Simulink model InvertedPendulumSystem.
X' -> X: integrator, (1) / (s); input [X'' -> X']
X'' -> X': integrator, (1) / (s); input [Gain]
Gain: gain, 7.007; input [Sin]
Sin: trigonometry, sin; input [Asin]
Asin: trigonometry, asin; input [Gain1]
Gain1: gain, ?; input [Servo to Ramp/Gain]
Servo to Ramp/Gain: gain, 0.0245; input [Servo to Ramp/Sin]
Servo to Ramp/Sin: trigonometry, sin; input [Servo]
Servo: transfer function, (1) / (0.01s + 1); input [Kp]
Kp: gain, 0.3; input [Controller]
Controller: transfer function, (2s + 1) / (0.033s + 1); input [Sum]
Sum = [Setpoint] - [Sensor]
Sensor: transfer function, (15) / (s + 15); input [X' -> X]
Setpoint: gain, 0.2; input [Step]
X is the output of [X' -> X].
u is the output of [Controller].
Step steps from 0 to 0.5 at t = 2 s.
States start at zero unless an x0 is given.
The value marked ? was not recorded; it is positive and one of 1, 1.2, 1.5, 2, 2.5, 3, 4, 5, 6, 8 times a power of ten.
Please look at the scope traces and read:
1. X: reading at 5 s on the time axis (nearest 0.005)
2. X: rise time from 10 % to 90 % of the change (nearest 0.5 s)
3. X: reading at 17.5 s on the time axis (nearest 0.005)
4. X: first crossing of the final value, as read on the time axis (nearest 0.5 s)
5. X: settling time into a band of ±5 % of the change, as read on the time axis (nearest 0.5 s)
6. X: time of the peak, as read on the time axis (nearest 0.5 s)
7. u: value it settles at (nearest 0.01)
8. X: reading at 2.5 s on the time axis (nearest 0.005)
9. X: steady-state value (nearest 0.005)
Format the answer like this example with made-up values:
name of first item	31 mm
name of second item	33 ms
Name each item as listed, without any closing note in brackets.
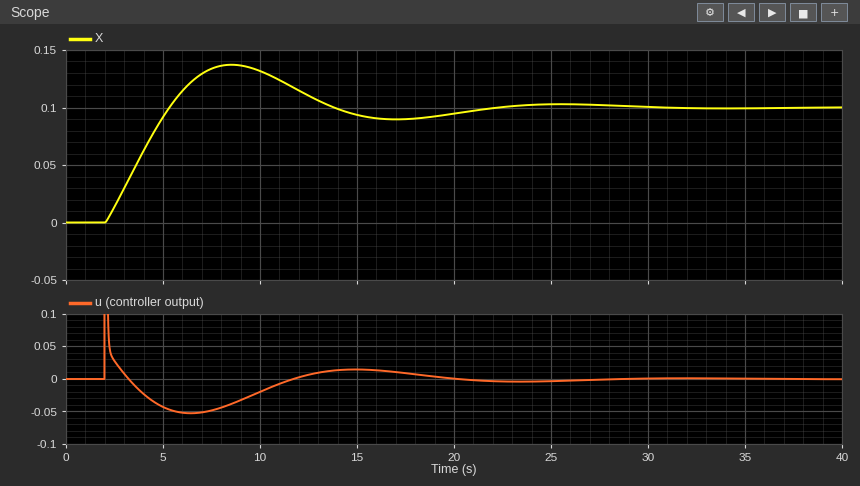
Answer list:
X: reading at 5 s on the time axis	0.090
X: rise time from 10 % to 90 % of the change	2.5 s
X: reading at 17.5 s on the time axis	0.090
X: first crossing of the final value, as read on the time axis	5.5 s
X: settling time into a band of ±5 % of the change, as read on the time axis	20.0 s
X: time of the peak, as read on the time axis	8.5 s
u: value it settles at	0.00
X: reading at 2.5 s on the time axis	0.015
X: steady-state value	0.100
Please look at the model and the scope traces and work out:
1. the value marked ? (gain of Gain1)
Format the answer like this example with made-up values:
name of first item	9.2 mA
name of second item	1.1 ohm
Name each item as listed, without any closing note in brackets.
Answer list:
the value marked ?	3
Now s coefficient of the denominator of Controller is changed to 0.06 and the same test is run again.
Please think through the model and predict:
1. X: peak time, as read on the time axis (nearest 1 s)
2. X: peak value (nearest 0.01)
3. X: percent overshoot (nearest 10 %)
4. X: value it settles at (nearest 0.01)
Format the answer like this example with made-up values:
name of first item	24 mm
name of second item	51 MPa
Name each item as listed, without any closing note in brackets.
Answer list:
X: peak time, as read on the time axis	8 s
X: peak value	0.14
X: percent overshoot	40 %
X: value it settles at	0.10
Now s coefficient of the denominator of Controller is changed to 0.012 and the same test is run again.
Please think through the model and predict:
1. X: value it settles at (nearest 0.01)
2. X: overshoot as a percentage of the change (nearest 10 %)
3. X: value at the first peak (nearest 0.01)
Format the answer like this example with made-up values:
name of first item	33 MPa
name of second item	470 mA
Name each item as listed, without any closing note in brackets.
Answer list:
X: value it settles at	0.10
X: overshoot as a percentage of the change	30 %
X: value at the first peak	0.13
